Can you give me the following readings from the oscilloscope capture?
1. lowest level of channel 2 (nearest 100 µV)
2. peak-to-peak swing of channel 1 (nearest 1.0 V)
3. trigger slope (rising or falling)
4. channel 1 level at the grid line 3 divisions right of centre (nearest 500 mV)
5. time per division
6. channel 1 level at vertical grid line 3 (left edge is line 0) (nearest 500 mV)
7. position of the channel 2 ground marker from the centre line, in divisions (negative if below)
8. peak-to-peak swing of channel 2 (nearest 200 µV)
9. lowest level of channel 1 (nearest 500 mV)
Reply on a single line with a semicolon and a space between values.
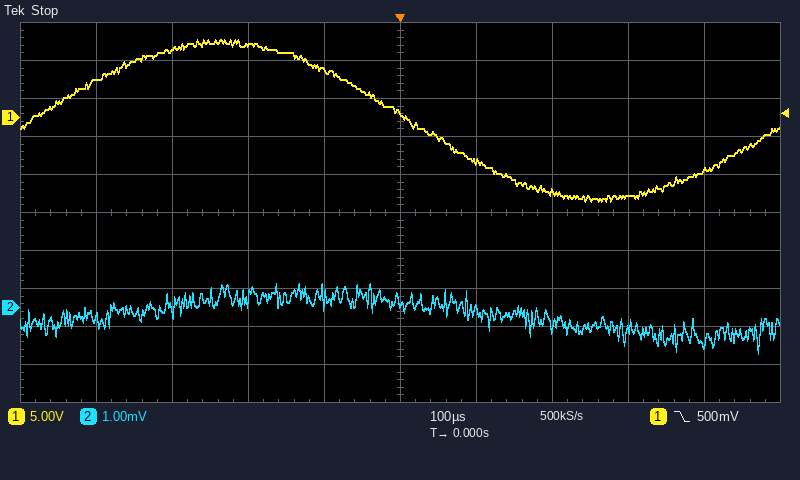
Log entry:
-1.2 mV; 21.0 V; falling; -10.5 V; 100 µs; 9.5 V; -2.5 div; 1.8 mV; -11.0 V
